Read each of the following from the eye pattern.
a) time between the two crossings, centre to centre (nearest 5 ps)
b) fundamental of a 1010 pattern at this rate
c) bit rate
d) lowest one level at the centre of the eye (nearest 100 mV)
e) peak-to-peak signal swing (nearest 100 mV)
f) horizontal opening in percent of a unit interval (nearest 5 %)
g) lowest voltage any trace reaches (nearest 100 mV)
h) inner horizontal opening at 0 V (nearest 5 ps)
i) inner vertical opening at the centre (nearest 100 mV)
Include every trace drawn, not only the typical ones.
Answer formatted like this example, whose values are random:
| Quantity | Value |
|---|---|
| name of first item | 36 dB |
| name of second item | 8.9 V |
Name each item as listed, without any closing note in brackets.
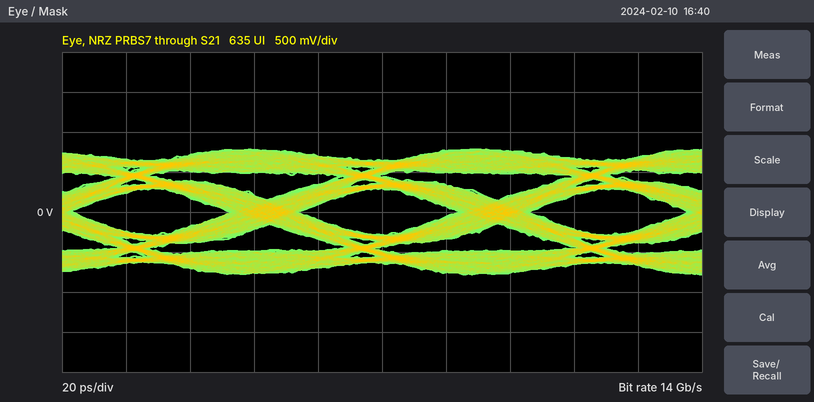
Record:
| Quantity | Value |
|---|---|
| time between the two crossings, centre to centre | 70 ps |
| fundamental of a 1010 pattern at this rate | 7 GHz |
| bit rate | 14 Gb/s |
| lowest one level at the centre of the eye | 300 mV |
| peak-to-peak signal swing | 1.6 V |
| horizontal opening in percent of a unit interval | 70 % |
| lowest voltage any trace reaches | -800 mV |
| inner horizontal opening at 0 V | 50 ps |
| inner vertical opening at the centre | 600 mV |
